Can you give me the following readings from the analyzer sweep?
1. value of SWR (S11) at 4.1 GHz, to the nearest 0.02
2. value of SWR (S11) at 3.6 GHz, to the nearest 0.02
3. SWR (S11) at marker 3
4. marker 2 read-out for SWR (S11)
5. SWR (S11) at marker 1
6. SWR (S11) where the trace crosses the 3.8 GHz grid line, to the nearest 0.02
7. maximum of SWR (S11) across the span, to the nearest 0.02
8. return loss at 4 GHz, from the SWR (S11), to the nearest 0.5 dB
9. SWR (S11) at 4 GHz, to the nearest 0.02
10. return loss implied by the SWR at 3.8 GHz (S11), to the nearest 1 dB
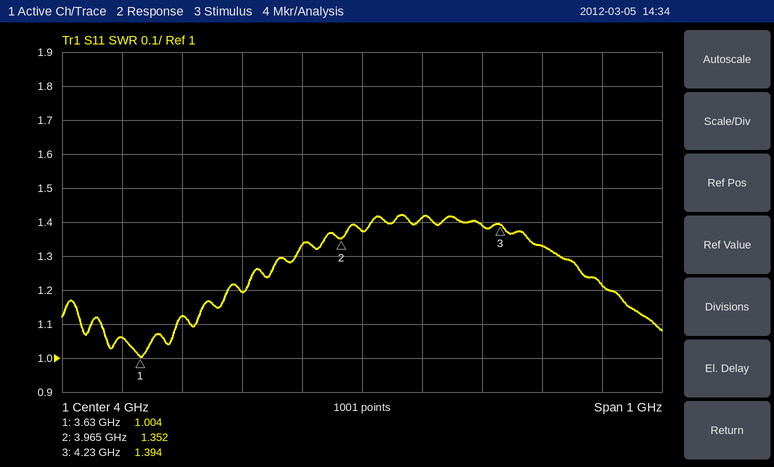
1.42
1.06
1.394
1.352
1.004
1.20
1.42
16.0 dB
1.38
21 dB
